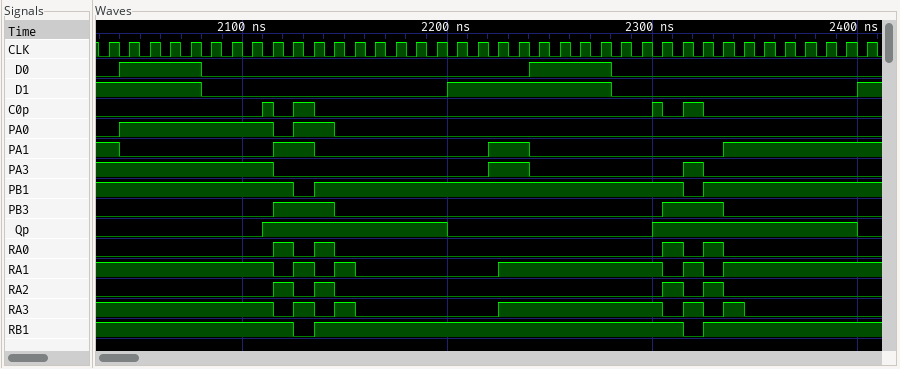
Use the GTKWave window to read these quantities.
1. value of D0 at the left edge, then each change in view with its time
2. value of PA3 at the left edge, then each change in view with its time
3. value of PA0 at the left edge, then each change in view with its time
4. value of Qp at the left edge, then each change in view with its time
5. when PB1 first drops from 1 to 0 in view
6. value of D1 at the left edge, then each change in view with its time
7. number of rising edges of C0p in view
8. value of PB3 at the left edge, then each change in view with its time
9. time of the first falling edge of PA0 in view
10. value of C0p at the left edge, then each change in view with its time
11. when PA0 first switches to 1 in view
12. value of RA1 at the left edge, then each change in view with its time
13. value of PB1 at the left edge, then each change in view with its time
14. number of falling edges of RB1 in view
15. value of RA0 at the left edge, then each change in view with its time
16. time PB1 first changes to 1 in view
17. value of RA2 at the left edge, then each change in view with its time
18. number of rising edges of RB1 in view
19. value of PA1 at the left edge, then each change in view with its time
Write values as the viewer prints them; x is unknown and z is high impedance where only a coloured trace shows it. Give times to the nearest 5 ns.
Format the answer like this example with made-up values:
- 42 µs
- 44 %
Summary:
- 0, 1 at 2040 ns, 0 at 2080 ns, 1 at 2240 ns, 0 at 2280 ns
- 1, 0 at 2115 ns, 1 at 2220 ns, 0 at 2240 ns, 1 at 2315 ns, 0 at 2325 ns
- 0, 1 at 2040 ns, 0 at 2115 ns, 1 at 2125 ns, 0 at 2145 ns
- 0, 1 at 2110 ns, 0 at 2200 ns, 1 at 2300 ns, 0 at 2400 ns
- 2125 ns
- 1, 0 at 2080 ns, 1 at 2200 ns, 0 at 2280 ns, 1 at 2400 ns
- 4
- 0, 1 at 2115 ns, 0 at 2145 ns, 1 at 2305 ns, 0 at 2335 ns
- 2115 ns
- 0, 1 at 2110 ns, 0 at 2115 ns, 1 at 2125 ns, 0 at 2135 ns, 1 at 2300 ns, 0 at 2305 ns, 1 at 2315 ns, 0 at 2325 ns
- 2040 ns
- 1, 0 at 2115 ns, 1 at 2125 ns, 0 at 2135 ns, 1 at 2145 ns, 0 at 2155 ns, 1 at 2225 ns, 0 at 2305 ns, 1 at 2315 ns, 0 at 2325 ns, 1 at 2335 ns
- 1, 0 at 2125 ns, 1 at 2135 ns, 0 at 2315 ns, 1 at 2325 ns
- 2
- 0, 1 at 2115 ns, 0 at 2125 ns, 1 at 2135 ns, 0 at 2145 ns, 1 at 2305 ns, 0 at 2315 ns, 1 at 2325 ns, 0 at 2335 ns
- 2135 ns
- 0, 1 at 2115 ns, 0 at 2125 ns, 1 at 2135 ns, 0 at 2145 ns, 1 at 2305 ns, 0 at 2315 ns, 1 at 2325 ns, 0 at 2335 ns
- 2
- 1, 0 at 2040 ns, 1 at 2115 ns, 0 at 2135 ns, 1 at 2220 ns, 0 at 2240 ns, 1 at 2335 ns
